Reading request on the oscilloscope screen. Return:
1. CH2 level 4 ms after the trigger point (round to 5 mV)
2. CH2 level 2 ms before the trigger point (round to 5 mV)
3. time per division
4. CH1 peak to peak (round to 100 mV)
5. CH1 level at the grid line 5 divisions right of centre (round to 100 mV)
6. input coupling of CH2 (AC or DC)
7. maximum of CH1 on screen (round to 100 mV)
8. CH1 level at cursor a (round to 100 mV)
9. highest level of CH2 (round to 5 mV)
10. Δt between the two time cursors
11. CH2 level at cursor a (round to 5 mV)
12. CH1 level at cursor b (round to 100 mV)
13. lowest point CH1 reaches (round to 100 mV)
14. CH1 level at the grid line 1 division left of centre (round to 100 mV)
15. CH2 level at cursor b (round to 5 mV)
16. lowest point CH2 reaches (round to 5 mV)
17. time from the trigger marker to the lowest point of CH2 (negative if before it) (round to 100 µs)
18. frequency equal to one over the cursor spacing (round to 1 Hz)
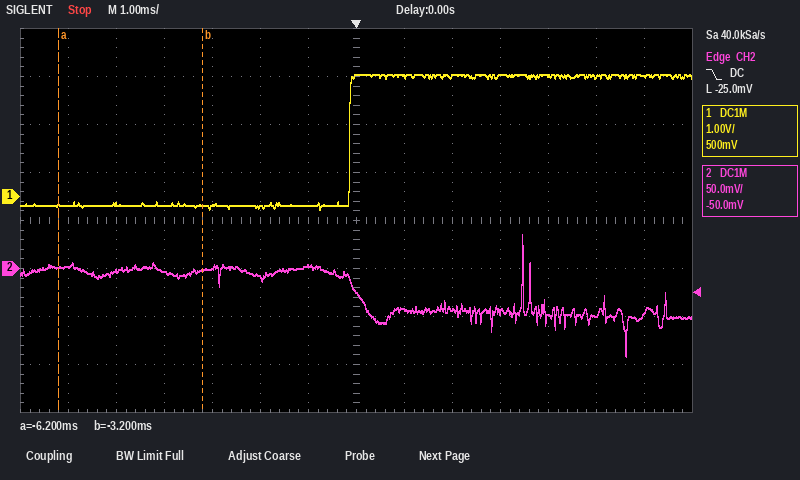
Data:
-50 mV
-10 mV
1 ms
2.8 V
2.5 V
DC
2.5 V
-200 mV
35 mV
3.0 ms
0 mV
-200 mV
-300 mV
-200 mV
0 mV
-90 mV
+5.6 ms
333 Hz
